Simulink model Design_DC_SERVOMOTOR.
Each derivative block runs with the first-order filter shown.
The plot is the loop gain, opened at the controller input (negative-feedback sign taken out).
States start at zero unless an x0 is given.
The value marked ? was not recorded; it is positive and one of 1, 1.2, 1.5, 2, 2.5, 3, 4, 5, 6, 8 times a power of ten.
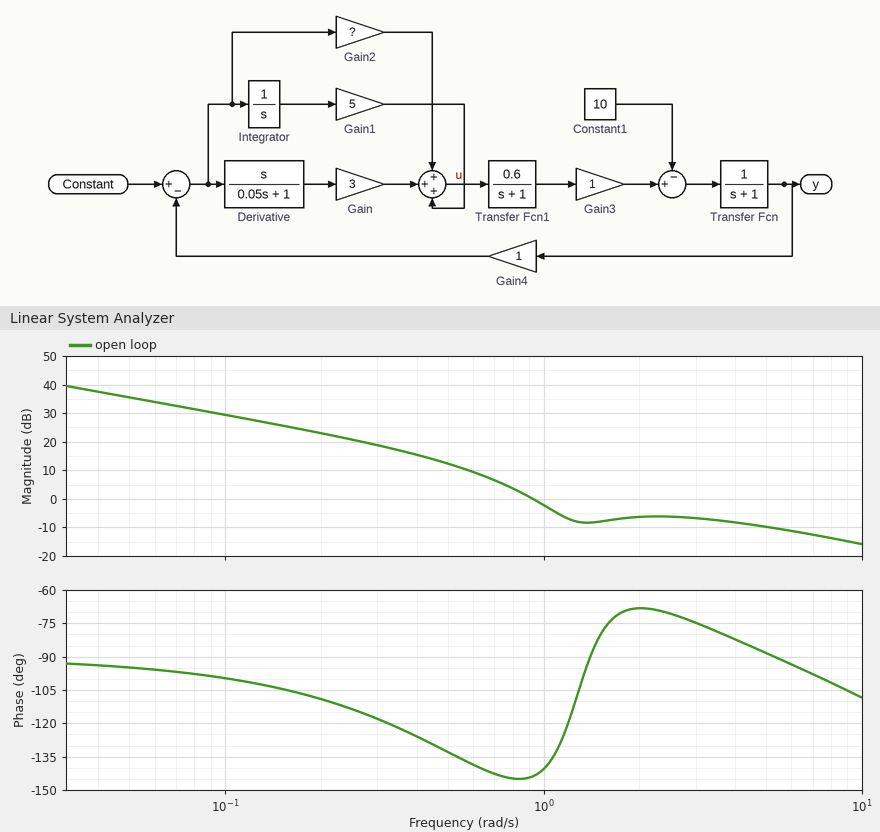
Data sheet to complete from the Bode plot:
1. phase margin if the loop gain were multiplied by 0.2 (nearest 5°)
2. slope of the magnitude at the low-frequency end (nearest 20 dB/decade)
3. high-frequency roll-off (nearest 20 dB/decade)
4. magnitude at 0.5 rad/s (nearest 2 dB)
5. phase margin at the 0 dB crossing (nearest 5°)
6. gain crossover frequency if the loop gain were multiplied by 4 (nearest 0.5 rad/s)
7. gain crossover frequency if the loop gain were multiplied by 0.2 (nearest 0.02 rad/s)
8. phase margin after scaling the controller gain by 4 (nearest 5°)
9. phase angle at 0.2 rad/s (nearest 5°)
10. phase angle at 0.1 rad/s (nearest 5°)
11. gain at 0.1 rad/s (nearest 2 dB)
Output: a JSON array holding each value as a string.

["50°", "-20 dB/decade", "-20 dB/decade", "12 dB", "35°", "6.5 rad/s", "0.44 rad/s", "85°", "-110°", "-100°", "30 dB"]
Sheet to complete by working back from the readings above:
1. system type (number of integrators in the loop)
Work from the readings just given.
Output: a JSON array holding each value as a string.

["1"]
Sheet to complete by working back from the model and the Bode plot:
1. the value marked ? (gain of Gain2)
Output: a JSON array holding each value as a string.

["1.5"]
